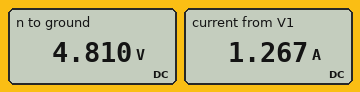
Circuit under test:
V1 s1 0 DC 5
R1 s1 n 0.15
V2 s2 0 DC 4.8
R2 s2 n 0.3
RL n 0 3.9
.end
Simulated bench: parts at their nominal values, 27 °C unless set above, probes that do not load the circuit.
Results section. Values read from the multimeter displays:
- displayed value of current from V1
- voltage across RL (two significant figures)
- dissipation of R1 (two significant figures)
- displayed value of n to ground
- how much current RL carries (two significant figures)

1.267 A
4.8 V
240 mW
4.810 V
1.2 A
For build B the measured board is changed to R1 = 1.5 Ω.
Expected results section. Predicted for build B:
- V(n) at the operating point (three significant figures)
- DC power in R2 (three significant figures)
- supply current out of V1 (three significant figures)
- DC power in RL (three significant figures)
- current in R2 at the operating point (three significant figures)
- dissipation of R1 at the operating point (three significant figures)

4.54 V
222 mW
305 mA
5.29 W
859 mA
140 mW
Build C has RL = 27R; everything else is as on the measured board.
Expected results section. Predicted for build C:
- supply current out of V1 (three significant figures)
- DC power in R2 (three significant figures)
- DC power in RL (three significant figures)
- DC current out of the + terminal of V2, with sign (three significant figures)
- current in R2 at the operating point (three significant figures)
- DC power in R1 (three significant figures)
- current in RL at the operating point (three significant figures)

566 mA
44.2 mW
895 mW
-384 mA
384 mA
48.0 mW
182 mA
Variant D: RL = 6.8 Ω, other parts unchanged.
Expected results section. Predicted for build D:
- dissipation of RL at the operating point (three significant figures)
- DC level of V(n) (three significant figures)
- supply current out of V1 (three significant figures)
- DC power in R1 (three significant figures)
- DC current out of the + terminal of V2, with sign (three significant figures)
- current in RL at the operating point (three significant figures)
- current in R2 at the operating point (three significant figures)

3.48 W
4.86 V
921 mA
127 mW
-206 mA
715 mA
206 mA
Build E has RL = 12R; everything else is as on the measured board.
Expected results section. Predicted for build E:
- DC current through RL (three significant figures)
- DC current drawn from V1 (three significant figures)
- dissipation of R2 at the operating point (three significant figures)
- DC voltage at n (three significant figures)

408 mA
716 mA
28.6 mW
4.89 V
